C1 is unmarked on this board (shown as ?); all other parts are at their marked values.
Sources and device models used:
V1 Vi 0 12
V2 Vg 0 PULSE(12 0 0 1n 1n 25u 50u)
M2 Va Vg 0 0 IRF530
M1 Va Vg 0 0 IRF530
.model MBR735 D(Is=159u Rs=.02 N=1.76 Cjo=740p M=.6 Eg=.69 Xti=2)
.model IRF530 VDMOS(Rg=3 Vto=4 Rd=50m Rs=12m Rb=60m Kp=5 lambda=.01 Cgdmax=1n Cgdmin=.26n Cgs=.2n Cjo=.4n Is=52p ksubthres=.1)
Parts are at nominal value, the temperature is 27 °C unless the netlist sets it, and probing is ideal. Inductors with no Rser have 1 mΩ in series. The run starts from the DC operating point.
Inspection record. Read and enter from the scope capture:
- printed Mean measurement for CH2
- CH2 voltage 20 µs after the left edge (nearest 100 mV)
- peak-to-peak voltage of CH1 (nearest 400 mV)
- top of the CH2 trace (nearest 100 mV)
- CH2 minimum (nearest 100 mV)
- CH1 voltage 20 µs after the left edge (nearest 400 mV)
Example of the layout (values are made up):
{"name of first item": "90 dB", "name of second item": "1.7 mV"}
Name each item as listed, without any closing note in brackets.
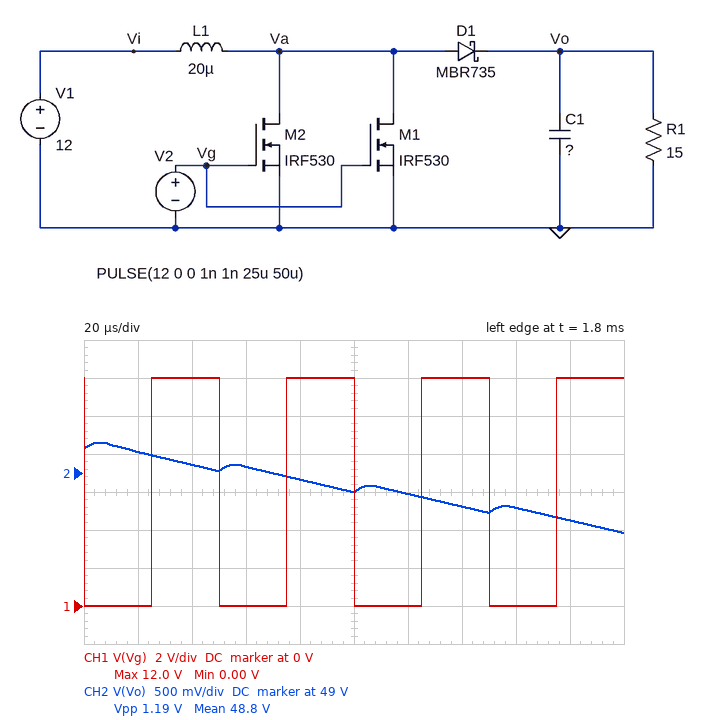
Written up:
{"printed Mean measurement for CH2": "48.8 V", "CH2 voltage 20 µs after the left edge": "49.3 V", "peak-to-peak voltage of CH1": "12.0 V", "top of the CH2 trace": "49.4 V", "CH2 minimum": "48.2 V", "CH1 voltage 20 µs after the left edge": "0 V"}
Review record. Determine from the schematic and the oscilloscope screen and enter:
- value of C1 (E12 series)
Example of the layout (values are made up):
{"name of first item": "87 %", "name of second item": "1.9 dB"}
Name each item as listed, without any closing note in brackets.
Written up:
{"value of C1": "390 µF"}
